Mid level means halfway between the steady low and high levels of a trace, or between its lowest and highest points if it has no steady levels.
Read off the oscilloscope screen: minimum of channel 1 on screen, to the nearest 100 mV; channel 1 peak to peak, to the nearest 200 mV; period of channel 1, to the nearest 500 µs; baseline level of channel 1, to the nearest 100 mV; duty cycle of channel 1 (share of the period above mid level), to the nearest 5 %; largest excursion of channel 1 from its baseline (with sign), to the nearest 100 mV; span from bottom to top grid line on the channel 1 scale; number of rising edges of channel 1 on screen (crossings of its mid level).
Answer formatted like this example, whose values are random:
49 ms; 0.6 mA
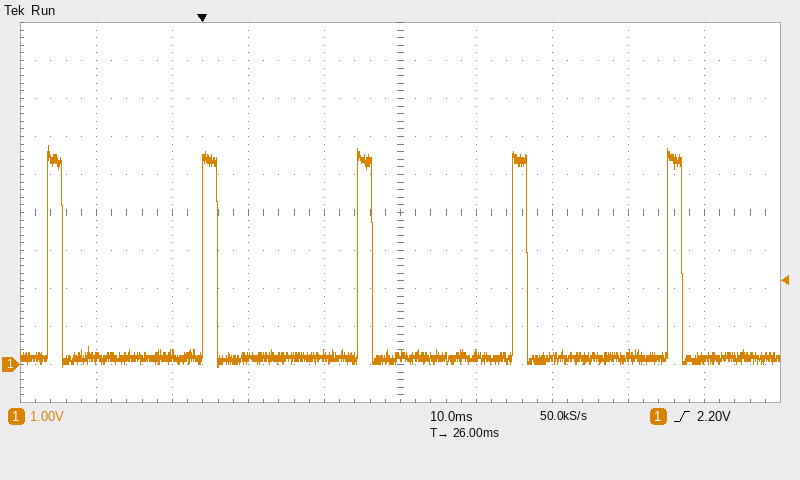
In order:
-100 mV; 5.8 V; 20.5 ms; 200 mV; 10 %; +5.6 V; 10 V; 5
